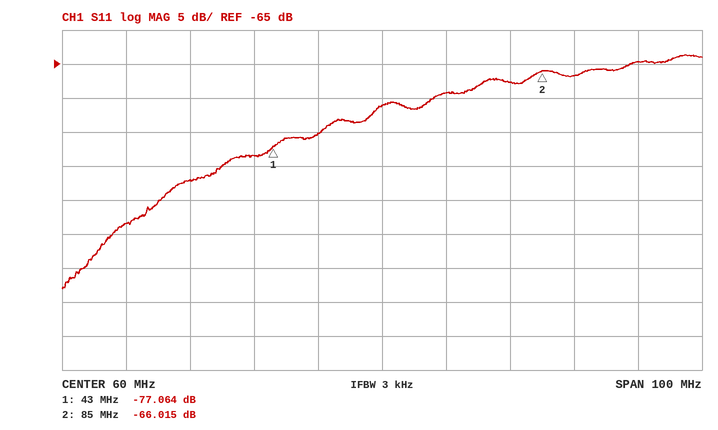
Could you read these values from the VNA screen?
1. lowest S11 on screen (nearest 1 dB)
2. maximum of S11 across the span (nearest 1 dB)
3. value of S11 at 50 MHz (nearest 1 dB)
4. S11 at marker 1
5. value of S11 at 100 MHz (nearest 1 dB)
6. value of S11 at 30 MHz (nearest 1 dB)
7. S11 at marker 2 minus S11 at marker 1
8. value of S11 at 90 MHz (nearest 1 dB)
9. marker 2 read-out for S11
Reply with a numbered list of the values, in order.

1. -98 dB
2. -64 dB
3. -75 dB
4. -77.064 dB
5. -65 dB
6. -82 dB
7. 11.049 dB
8. -67 dB
9. -66.015 dB
